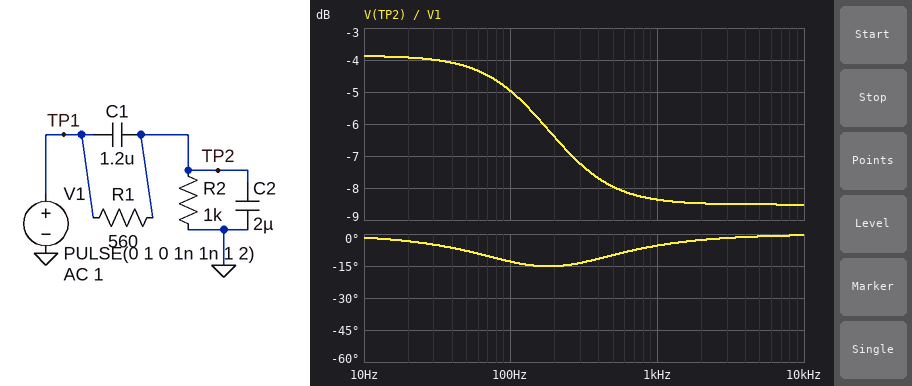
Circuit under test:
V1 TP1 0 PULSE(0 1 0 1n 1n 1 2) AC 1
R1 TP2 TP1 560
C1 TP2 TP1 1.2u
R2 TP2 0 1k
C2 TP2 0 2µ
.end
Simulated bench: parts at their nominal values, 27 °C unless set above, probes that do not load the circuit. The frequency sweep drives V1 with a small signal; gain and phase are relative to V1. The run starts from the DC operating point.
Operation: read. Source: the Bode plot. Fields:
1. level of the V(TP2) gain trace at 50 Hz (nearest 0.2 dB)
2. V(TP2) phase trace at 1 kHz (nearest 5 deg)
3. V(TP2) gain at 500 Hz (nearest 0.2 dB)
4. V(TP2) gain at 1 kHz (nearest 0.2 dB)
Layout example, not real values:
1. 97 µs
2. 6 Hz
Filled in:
1. -4.2 dB
2. -5 deg
3. -8.0 dB
4. -8.4 dB
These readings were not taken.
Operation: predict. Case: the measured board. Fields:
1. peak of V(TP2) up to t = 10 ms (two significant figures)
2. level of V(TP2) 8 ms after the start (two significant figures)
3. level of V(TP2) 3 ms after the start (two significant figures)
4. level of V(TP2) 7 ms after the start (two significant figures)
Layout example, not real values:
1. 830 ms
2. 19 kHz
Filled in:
1. 640 mV
2. 640 mV
3. 620 mV
4. 640 mV
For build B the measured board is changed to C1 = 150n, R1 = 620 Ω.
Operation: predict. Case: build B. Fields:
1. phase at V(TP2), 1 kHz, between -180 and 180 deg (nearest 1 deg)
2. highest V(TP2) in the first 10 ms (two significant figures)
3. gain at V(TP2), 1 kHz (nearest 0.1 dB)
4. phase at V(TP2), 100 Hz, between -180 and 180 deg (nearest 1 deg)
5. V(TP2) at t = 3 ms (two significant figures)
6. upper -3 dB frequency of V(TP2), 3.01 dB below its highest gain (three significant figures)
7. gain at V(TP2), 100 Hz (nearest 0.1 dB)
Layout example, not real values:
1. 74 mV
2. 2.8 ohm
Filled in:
1. -49 deg
2. 620 mV
3. -17.3 dB
4. -24 deg
5. 600 mV
6. 196 Hz
7. -5.2 dB
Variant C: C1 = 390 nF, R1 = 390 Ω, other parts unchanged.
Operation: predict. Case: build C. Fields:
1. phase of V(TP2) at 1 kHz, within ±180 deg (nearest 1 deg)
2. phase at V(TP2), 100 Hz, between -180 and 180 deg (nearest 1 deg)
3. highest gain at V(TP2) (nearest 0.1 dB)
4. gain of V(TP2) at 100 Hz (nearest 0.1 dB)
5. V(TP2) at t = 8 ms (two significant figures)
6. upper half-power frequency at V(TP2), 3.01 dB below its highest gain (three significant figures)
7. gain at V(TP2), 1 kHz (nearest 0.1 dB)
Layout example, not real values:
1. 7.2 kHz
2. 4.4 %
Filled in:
1. -33 deg
2. -17 deg
3. -2.9 dB
4. -3.5 dB
5. 720 mV
6. 251 Hz
7. -12.8 dB
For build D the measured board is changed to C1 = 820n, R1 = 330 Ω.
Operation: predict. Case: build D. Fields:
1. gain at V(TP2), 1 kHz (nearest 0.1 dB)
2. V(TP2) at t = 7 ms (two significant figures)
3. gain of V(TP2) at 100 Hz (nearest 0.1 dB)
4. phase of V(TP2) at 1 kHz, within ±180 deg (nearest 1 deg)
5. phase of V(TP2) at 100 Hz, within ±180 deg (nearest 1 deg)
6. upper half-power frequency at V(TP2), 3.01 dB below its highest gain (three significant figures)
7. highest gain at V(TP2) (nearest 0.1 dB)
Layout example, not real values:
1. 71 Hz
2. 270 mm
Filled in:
1. -9.7 dB
2. 750 mV
3. -3.1 dB
4. -18 deg
5. -14 deg
6. 272 Hz
7. -2.5 dB
